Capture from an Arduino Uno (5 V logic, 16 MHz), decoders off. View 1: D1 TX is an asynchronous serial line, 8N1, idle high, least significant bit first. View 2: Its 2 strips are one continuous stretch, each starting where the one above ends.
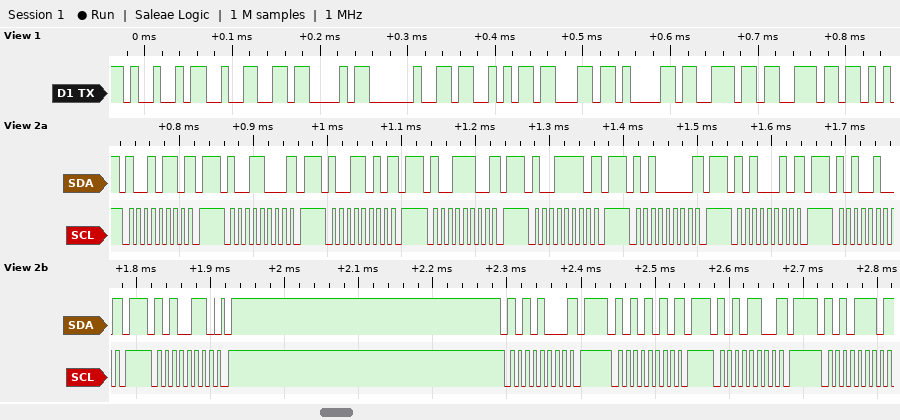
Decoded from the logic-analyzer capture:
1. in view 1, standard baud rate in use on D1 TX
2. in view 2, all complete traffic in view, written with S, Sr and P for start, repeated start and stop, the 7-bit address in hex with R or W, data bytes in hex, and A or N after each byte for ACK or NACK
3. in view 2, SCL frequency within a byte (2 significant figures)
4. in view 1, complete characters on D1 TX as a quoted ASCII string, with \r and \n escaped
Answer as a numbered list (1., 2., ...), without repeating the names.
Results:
1. 115200 baud
2. S 4BW N P S 4CW N P S 4DW N P S 4EW N P S 4FW N P S 50W N P S 51W N P S 52W N P S 53W A P S 54W N P S 55W N P S 56W N P S 57W N
3. 100 kHz
4. "I2C Scann"
